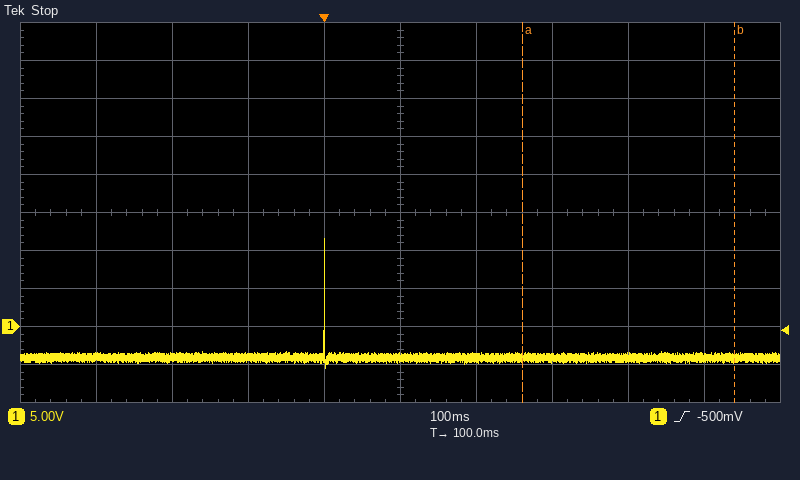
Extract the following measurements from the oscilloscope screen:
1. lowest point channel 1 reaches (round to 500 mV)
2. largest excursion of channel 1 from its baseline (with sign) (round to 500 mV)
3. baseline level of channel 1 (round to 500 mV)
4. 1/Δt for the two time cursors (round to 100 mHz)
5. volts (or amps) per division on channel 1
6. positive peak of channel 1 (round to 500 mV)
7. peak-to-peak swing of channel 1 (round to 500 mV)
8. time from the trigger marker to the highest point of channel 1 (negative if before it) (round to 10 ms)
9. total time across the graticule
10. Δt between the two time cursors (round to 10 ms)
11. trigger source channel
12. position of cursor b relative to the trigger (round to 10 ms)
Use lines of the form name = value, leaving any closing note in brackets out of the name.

lowest point channel 1 reaches = -5.5 V
largest excursion of channel 1 from its baseline (with sign) = +15.5 V
baseline level of channel 1 = -4.0 V
1/Δt for the two time cursors = 3.6 Hz
volts (or amps) per division on channel 1 = 5 V
positive peak of channel 1 = 11.5 V
peak-to-peak swing of channel 1 = 17.0 V
time from the trigger marker to the highest point of channel 1 (negative if before it) = 0 ms
total time across the graticule = 1 s
Δt between the two time cursors = 280 ms
trigger source channel = channel 1
position of cursor b relative to the trigger = +540 ms
